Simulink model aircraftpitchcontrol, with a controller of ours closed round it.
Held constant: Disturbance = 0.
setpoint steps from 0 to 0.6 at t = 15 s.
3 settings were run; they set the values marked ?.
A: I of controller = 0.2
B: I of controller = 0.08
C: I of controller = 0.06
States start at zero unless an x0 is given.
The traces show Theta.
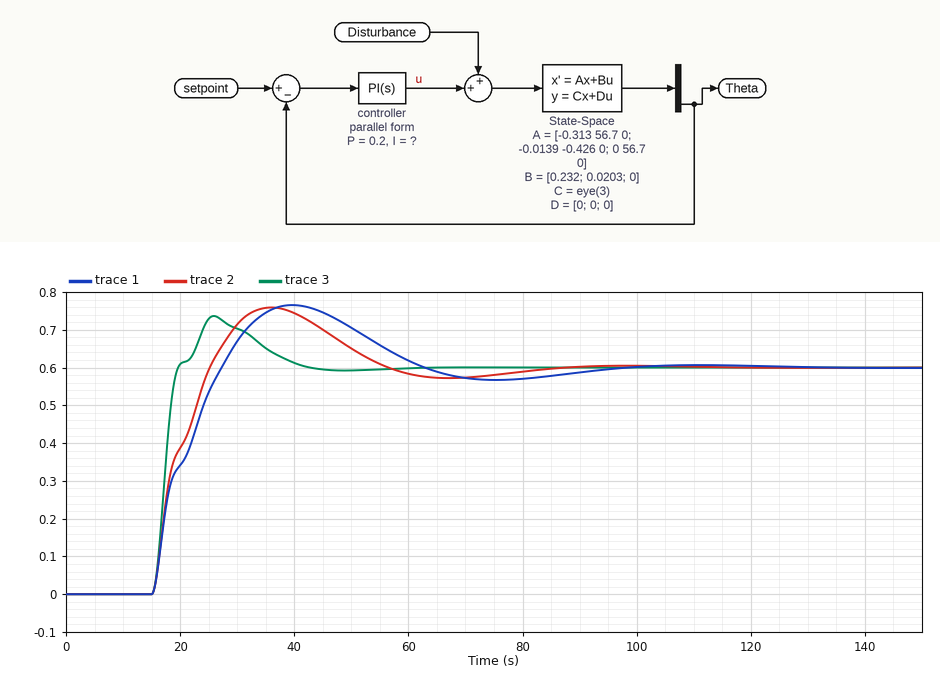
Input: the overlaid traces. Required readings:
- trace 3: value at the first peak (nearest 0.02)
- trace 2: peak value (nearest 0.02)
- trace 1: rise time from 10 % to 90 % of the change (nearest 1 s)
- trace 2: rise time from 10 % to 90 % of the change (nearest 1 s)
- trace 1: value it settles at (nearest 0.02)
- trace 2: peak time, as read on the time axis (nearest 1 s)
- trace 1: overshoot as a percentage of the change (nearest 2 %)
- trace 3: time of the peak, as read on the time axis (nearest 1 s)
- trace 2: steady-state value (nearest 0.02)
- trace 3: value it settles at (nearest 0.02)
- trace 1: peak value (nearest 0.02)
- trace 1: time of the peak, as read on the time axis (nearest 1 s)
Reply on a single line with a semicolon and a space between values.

0.74; 0.76; 9 s; 8 s; 0.60; 36 s; 28 %; 26 s; 0.60; 0.60; 0.76; 40 s
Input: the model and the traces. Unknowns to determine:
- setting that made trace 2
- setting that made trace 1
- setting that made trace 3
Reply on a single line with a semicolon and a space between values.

B; C; A
